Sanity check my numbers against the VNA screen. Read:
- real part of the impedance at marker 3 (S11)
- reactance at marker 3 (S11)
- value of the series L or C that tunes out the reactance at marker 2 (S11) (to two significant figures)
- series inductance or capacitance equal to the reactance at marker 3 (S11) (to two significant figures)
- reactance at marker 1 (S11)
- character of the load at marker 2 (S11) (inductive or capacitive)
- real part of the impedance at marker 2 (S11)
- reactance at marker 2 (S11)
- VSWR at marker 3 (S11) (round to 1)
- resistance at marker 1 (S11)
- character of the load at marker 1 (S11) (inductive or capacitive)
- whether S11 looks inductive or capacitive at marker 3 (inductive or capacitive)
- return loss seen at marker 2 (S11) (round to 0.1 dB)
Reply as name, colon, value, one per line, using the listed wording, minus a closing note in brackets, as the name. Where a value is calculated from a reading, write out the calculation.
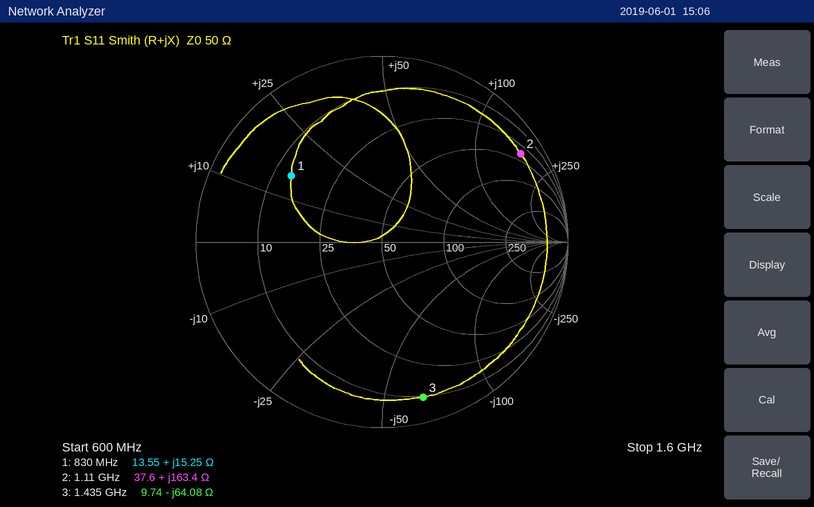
real part of the impedance at marker 3: 9.74 Ω
reactance at marker 3: -64.08 Ω
value of the series L or C that tunes out the reactance at marker 2 (S11): C = 1/(2π × 1.11 GHz × 163.4 Ω) ≈ 877 fF, so 880 fF to two significant figures
series inductance or capacitance equal to the reactance at marker 3 (S11): C = 1/(2π × 1.435 GHz × 64.08 Ω) ≈ 1.7 pF
reactance at marker 1: +15.25 Ω
character of the load at marker 2 (S11): inductive
real part of the impedance at marker 2: 37.6 Ω
reactance at marker 2: +163.4 Ω
VSWR at marker 3 (S11): 14
resistance at marker 1: 13.55 Ω
character of the load at marker 1 (S11): inductive
whether S11 looks inductive or capacitive at marker 3: capacitive
return loss seen at marker 2 (S11): 1.1 dB
